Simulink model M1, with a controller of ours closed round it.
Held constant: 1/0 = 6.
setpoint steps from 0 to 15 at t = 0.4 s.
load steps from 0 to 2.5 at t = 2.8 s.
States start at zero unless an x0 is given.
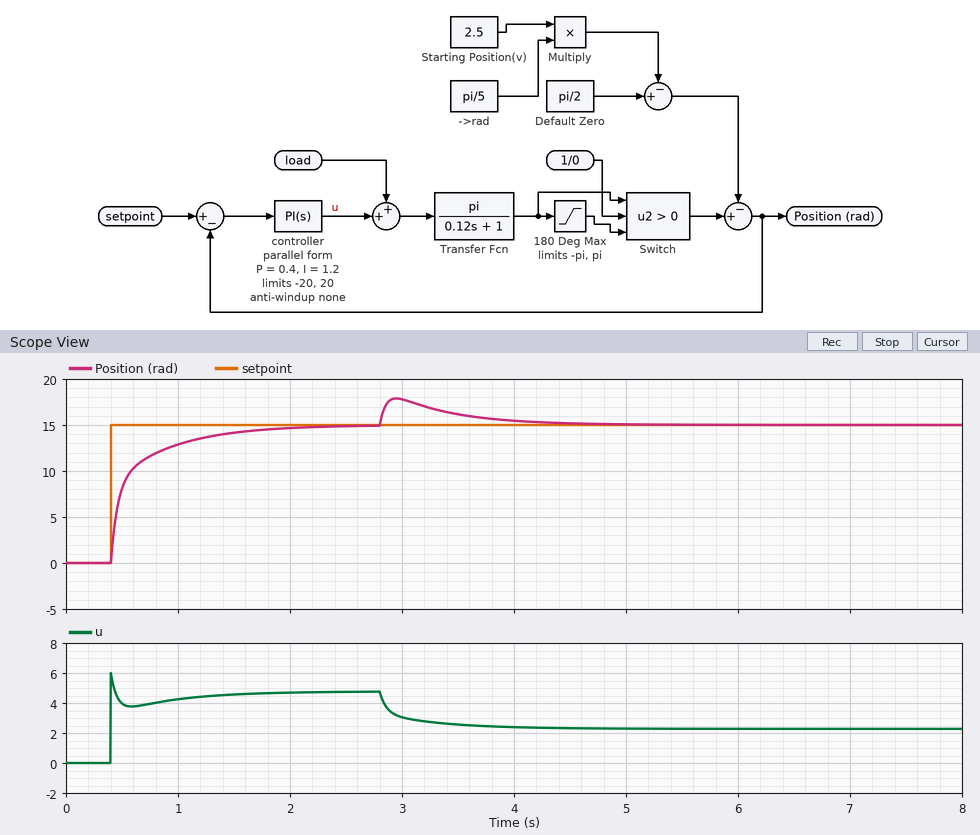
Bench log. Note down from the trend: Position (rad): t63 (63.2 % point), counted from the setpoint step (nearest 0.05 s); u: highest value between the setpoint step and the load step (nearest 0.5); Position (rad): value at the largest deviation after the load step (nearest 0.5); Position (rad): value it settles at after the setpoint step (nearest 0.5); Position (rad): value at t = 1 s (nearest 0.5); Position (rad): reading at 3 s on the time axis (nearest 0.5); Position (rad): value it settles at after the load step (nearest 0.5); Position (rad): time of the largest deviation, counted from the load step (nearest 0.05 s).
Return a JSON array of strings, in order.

["0.15 s", "6.0", "18.0", "15.0", "13.0", "18.0", "15.0", "0.15 s"]
